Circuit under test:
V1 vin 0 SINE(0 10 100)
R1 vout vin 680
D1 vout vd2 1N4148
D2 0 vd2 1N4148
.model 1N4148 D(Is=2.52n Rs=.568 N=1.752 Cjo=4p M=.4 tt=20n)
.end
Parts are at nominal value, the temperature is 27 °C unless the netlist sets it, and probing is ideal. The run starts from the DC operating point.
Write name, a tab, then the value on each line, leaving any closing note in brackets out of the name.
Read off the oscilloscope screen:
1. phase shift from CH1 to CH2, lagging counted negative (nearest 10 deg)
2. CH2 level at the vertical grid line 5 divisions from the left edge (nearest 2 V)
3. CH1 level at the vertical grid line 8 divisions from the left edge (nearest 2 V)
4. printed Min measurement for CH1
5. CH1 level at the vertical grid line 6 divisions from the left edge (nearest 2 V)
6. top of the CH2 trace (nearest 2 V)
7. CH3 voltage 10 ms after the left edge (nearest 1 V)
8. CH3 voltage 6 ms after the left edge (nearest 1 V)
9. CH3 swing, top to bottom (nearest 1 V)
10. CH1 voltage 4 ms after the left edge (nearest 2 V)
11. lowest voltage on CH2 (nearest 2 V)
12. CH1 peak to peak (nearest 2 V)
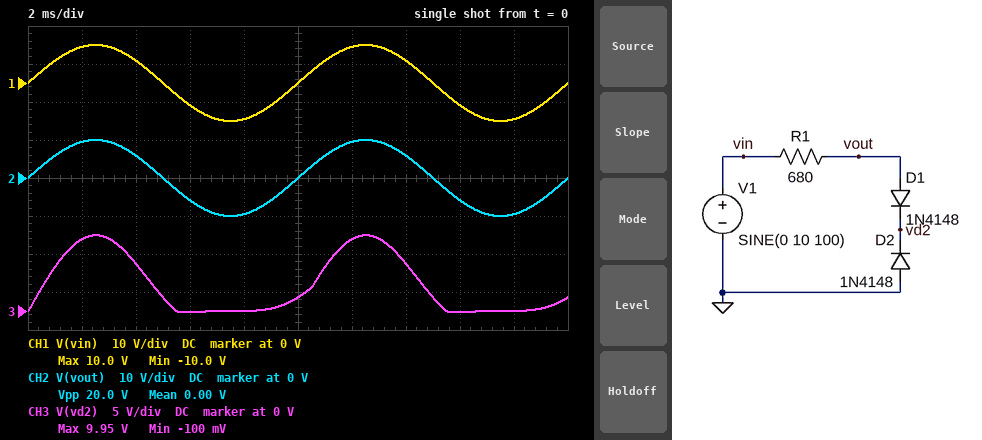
phase shift from CH1 to CH2, lagging counted negative	0 deg
CH2 level at the vertical grid line 5 divisions from the left edge	0 V
CH1 level at the vertical grid line 8 divisions from the left edge	-6 V
printed Min measurement for CH1	-10.0 V
CH1 level at the vertical grid line 6 divisions from the left edge	10 V
top of the CH2 trace	10 V
CH3 voltage 10 ms after the left edge	2 V
CH3 voltage 6 ms after the left edge	0 V
CH3 swing, top to bottom	10 V
CH1 voltage 4 ms after the left edge	6 V
lowest voltage on CH2	-10 V
CH1 peak to peak	20 V
